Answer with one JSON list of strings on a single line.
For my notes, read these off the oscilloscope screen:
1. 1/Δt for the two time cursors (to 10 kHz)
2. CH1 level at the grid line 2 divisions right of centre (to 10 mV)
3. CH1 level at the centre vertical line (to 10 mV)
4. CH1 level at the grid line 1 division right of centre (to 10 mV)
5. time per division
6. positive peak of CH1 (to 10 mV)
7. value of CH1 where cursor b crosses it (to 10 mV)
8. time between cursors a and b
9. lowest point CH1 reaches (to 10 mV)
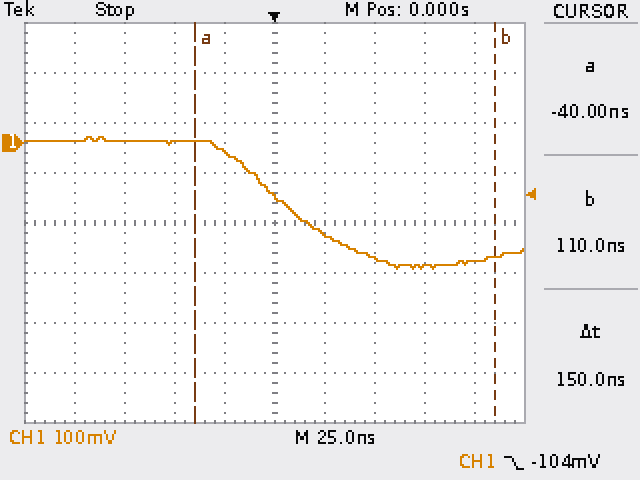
["6.67 MHz", "-230 mV", "-110 mV", "-180 mV", "25 ns", "10 mV", "-230 mV", "150 ns", "-250 mV"]
